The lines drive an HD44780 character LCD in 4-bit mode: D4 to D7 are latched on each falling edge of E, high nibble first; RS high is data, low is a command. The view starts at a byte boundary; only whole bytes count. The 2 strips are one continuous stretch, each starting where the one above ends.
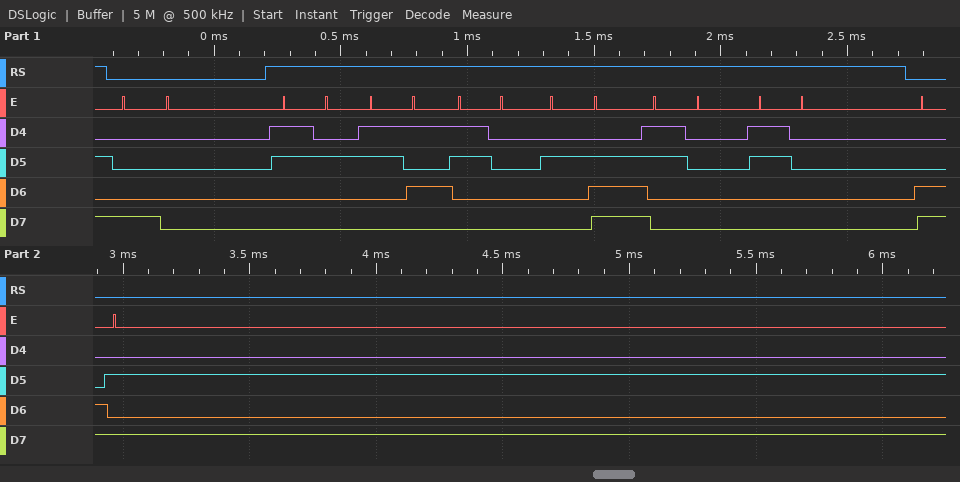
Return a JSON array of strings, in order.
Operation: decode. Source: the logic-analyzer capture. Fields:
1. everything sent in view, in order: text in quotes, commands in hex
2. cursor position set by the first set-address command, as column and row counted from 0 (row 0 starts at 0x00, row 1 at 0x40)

["0x80 \"250.00\" 0xCA", "column 0, row 0"]
